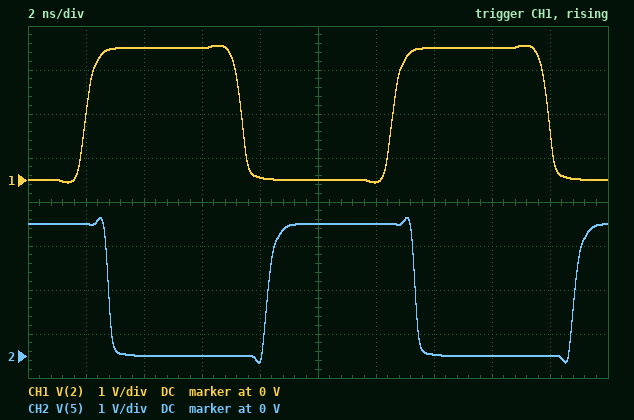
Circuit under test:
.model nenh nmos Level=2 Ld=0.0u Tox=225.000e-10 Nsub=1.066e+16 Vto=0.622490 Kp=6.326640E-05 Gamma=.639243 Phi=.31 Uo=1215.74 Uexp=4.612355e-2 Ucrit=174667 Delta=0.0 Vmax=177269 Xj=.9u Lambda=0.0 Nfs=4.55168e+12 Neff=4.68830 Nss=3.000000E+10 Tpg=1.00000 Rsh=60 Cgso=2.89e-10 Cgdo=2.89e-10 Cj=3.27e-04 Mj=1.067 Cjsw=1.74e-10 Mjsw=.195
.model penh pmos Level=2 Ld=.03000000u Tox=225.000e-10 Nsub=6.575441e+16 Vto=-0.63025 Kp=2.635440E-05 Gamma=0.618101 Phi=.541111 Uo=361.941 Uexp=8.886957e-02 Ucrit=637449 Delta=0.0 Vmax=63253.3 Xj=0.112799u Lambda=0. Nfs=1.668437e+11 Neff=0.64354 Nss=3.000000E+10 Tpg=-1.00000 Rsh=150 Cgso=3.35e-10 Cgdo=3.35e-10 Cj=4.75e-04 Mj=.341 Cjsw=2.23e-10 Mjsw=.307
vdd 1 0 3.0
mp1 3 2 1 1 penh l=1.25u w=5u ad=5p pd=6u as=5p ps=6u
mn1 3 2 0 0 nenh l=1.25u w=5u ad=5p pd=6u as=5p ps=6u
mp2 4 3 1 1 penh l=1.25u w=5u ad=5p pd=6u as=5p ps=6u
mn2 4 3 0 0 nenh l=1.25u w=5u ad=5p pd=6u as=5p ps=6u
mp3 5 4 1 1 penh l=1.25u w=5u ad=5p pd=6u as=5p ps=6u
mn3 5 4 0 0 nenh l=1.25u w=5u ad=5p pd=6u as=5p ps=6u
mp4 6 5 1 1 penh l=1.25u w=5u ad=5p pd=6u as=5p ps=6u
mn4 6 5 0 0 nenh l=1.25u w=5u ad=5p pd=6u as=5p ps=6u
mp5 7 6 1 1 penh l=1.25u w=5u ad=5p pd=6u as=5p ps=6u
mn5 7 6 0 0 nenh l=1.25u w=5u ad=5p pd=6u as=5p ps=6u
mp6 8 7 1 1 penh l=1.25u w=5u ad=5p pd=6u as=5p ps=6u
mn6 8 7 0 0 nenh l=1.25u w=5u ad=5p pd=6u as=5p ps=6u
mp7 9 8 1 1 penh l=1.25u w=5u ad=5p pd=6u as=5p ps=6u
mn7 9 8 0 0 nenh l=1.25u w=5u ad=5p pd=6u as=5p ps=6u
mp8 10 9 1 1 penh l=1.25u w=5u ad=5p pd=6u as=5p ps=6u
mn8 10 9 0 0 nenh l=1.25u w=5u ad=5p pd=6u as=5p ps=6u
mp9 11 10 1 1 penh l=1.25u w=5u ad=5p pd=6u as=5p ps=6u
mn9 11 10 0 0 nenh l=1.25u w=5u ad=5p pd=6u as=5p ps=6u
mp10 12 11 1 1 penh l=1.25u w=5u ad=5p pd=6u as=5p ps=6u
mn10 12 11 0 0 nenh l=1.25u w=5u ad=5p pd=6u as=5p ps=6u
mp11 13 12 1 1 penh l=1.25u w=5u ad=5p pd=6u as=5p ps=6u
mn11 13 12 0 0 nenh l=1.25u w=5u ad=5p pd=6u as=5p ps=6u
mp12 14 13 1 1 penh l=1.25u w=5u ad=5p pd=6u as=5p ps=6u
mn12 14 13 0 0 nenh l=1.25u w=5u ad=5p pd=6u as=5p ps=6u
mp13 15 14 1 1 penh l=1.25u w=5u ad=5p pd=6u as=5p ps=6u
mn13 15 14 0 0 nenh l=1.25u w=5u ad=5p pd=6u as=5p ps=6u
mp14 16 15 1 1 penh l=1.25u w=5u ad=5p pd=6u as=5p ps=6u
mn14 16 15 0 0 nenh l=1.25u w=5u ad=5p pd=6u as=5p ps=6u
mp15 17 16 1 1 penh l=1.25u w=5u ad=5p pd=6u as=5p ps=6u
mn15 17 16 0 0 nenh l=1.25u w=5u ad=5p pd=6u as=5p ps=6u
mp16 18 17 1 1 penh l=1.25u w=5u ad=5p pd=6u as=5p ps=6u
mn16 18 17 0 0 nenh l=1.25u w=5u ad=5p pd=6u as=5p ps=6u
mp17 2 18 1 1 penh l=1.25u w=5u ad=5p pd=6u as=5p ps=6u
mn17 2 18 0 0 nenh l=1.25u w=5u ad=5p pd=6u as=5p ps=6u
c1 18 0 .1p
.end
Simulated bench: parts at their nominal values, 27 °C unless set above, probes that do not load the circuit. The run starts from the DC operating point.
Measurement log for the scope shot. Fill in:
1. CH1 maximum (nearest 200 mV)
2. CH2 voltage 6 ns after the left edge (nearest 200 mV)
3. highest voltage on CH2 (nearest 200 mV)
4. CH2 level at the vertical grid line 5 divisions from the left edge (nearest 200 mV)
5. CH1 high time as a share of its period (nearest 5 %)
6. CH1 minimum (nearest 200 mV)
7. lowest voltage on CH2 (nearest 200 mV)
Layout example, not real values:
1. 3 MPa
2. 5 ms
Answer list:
1. 3.0 V
2. 0 V
3. 3.2 V
4. 3.0 V
5. 50 %
6. 0 V
7. -200 mV
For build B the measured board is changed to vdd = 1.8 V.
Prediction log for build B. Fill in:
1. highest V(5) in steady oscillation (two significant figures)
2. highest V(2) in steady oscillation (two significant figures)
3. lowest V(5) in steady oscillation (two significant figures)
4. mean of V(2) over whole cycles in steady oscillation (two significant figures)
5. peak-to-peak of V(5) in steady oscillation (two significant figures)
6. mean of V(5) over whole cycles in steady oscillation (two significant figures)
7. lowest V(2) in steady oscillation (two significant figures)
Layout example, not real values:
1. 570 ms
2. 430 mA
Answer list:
1. 1.9 V
2. 1.8 V
3. -130 mV
4. 910 mV
5. 2.0 V
6. 860 mV
7. -46 mV
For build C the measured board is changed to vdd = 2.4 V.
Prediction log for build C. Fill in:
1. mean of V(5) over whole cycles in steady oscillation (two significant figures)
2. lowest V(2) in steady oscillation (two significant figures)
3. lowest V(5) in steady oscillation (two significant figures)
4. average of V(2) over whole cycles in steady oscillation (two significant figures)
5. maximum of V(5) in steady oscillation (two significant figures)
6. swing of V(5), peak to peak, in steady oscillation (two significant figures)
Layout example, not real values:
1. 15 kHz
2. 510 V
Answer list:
1. 1.1 V
2. -51 mV
3. -140 mV
4. 1.2 V
5. 2.5 V
6. 2.7 V
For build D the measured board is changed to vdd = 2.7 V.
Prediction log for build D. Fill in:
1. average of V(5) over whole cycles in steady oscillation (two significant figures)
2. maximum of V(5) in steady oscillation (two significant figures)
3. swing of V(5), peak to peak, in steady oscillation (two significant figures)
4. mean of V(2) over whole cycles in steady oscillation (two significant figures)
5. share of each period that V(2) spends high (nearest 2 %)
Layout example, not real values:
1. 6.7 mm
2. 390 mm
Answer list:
1. 1.3 V
2. 2.8 V
3. 3.0 V
4. 1.4 V
5. 50 %
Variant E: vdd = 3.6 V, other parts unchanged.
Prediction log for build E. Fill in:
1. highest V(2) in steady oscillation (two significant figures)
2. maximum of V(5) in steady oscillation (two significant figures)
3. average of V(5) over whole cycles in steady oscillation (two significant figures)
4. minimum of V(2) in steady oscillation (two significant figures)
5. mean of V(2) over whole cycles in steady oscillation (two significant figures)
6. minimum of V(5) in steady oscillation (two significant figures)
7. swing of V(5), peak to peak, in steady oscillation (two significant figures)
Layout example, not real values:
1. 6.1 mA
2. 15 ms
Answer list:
1. 3.7 V
2. 3.8 V
3. 1.7 V
4. -65 mV
5. 1.8 V
6. -170 mV
7. 3.9 V
